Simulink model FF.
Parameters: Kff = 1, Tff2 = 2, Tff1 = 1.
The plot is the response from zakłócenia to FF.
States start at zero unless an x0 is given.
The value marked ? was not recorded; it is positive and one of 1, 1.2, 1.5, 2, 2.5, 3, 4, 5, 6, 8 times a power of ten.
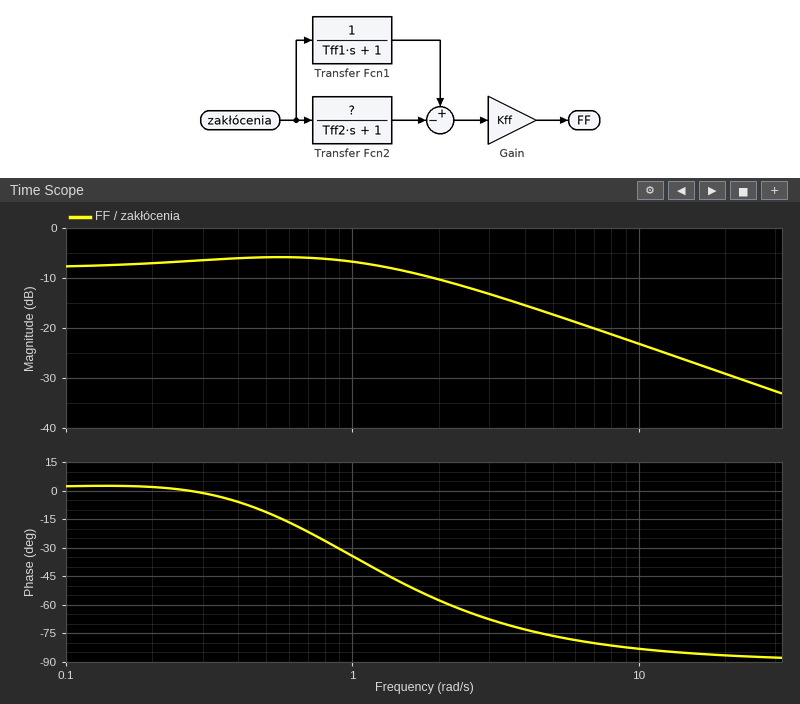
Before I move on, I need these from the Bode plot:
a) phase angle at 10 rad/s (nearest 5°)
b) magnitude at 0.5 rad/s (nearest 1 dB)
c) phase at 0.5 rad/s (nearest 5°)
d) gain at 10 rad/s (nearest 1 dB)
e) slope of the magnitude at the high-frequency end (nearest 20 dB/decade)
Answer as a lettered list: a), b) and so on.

a) -85°
b) -6 dB
c) -10°
d) -23 dB
e) -20 dB/decade
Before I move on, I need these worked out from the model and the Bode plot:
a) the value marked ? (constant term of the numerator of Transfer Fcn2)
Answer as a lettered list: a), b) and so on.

a) 0.6
